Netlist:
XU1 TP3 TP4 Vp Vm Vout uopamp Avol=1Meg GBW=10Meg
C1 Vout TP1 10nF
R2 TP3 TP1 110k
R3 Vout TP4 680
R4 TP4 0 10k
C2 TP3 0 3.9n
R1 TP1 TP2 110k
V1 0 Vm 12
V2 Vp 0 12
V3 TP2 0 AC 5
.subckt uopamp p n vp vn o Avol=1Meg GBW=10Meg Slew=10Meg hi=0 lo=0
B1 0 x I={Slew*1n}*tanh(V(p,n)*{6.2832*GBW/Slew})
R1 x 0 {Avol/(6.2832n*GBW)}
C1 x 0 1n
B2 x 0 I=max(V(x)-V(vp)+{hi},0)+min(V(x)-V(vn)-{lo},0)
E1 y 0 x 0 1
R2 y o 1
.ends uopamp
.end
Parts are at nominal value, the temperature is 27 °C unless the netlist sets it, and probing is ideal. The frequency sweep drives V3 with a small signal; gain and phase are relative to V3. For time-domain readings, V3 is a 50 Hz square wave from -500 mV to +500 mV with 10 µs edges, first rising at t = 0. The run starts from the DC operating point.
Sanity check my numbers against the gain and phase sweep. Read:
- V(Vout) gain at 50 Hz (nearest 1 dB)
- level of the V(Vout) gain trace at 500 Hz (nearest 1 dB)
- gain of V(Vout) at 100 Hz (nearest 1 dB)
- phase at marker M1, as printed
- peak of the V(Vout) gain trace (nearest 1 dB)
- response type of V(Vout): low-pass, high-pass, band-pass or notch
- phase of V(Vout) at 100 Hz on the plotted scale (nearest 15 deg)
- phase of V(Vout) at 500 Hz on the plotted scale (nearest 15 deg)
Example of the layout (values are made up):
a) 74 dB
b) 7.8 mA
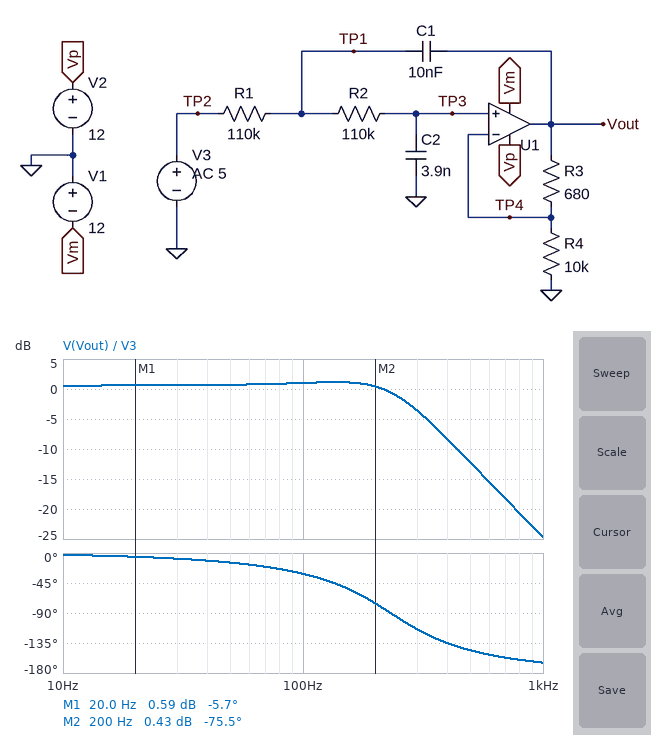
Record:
a) 1 dB
b) -12 dB
c) 1 dB
d) -5.7 deg
e) 1 dB
f) low-pass
g) -30 deg
h) -150 deg
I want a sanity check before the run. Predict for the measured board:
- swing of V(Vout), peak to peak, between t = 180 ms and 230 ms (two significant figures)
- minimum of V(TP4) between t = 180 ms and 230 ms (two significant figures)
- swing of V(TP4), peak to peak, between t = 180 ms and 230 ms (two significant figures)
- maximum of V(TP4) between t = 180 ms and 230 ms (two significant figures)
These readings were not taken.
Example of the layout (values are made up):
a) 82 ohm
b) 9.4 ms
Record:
a) 1.3 V
b) -610 mV
c) 1.2 V
d) 610 mV
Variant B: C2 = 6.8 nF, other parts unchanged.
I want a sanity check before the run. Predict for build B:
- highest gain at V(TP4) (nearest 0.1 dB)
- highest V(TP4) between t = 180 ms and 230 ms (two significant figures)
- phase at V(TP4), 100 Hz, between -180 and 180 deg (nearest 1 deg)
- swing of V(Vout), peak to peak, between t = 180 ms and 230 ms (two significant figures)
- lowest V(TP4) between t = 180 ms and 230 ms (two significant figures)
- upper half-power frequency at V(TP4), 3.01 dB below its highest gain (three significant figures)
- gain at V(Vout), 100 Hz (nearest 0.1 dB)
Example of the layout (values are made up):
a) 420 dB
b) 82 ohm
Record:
a) 0 dB
b) 520 mV
c) -53 deg
d) 1.1 V
e) -520 mV
f) 157 Hz
g) -0.4 dB
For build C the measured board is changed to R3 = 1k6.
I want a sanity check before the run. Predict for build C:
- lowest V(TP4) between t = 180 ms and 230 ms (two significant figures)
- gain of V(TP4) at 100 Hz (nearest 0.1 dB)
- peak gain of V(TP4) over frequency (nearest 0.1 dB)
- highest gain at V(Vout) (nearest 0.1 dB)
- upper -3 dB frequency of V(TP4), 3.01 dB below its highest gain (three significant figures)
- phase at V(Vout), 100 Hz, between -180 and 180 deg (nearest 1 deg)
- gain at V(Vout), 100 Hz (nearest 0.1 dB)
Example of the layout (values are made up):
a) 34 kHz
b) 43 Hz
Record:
a) -670 mV
b) 0.7 dB
c) 1.3 dB
d) 2.6 dB
e) 271 Hz
f) -28 deg
g) 2.0 dB
